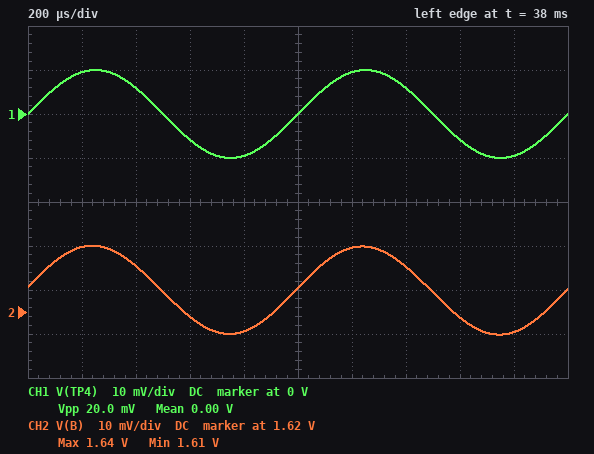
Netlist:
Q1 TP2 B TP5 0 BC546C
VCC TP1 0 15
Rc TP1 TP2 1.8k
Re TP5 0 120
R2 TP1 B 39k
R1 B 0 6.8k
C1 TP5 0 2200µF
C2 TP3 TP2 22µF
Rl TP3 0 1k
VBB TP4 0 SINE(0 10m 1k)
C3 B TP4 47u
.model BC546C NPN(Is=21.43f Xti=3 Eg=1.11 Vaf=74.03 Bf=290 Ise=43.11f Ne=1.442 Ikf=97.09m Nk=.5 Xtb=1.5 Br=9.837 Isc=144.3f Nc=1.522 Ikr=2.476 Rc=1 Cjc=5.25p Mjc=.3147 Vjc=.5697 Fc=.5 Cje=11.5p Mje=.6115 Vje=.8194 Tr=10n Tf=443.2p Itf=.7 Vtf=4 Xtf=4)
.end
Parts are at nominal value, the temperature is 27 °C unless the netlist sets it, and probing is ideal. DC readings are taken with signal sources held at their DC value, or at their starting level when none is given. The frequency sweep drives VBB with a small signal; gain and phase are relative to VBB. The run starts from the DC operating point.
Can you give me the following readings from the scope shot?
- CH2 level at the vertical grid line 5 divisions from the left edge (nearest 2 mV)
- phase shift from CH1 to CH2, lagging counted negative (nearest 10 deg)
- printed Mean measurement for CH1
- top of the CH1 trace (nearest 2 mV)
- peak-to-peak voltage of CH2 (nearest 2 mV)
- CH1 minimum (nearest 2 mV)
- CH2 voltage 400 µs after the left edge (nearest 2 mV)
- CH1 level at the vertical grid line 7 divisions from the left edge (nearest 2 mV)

1.626 V
0 deg
0.00 V
10 mV
20 mV
-10 mV
1.630 V
6 mV
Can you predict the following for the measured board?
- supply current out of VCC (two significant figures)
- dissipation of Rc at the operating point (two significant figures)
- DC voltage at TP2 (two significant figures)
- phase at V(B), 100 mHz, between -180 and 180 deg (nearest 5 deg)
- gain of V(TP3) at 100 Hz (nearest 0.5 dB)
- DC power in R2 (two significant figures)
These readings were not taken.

8.1 mA
110 mW
1.0 V
85 deg
17.0 dB
4.6 mW
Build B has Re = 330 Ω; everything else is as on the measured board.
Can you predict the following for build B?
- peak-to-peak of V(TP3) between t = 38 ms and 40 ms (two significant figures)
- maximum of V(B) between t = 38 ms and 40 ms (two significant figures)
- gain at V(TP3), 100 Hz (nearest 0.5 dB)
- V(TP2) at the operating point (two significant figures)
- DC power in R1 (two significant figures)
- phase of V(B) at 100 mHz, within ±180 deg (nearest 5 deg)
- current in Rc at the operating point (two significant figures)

2.0 V
2.1 V
40.0 dB
7.1 V
660 µW
80 deg
4.4 mA
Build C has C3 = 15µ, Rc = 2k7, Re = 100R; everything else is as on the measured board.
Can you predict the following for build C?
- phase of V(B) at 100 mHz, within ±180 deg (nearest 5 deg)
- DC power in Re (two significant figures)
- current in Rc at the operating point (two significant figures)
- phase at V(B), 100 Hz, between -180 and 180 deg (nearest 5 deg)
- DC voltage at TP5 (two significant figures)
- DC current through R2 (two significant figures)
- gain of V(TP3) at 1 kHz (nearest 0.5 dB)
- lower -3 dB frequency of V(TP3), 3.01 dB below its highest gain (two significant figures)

85 deg
3.0 mW
5.3 mA
70 deg
550 mV
350 µA
10.5 dB
270 Hz
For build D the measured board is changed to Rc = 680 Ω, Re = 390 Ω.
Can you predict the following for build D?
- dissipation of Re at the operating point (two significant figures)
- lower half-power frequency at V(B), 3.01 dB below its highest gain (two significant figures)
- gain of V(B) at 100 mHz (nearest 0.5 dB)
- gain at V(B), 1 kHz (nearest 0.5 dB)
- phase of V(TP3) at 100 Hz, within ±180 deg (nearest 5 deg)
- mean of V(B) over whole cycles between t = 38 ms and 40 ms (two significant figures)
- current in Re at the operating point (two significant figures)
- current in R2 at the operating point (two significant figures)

5.6 mW
790 mHz
-16.0 dB
0 dB
-170 deg
2.1 V
3.8 mA
330 µA
